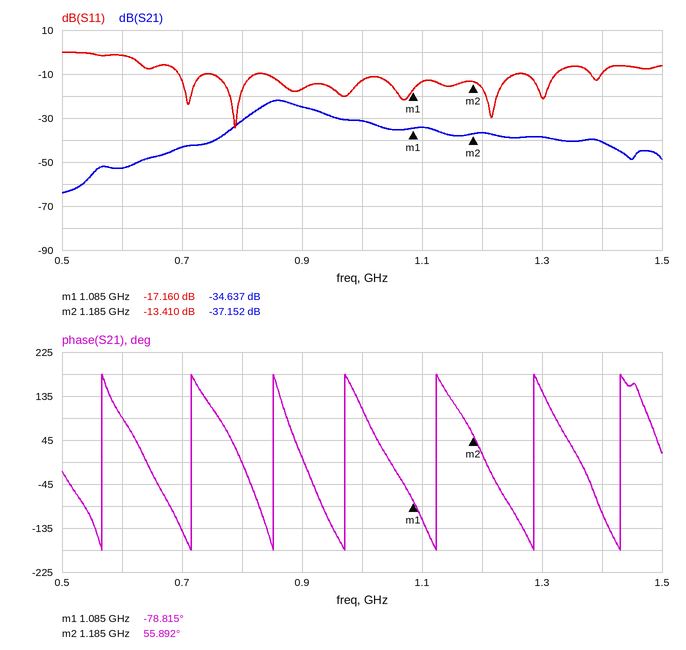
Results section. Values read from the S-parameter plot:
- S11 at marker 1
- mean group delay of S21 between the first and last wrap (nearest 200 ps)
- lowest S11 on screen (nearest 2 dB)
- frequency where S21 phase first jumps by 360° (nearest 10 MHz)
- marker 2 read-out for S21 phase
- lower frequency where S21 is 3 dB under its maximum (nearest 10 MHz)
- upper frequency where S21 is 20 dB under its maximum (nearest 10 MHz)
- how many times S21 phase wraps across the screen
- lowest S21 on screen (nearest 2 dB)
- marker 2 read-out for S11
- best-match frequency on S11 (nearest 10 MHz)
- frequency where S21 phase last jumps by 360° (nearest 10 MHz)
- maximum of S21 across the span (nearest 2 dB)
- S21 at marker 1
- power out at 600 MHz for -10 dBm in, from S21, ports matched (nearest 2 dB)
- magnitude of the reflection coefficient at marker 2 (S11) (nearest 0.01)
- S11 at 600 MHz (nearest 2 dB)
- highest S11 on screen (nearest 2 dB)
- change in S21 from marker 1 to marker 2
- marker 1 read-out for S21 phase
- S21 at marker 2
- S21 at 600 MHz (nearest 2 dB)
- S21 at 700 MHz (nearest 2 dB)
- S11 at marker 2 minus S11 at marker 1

-17.160 dB
7.0 ns
-34 dB
570 MHz
55.892°
830 MHz
1.41 GHz
7
-64 dB
-13.410 dB
790 MHz
1.43 GHz
-22 dB
-34.637 dB
-62 dBm
0.21
-2 dB
0 dB
-2.515 dB
-78.815°
-37.152 dB
-52 dB
-44 dB
3.750 dB
